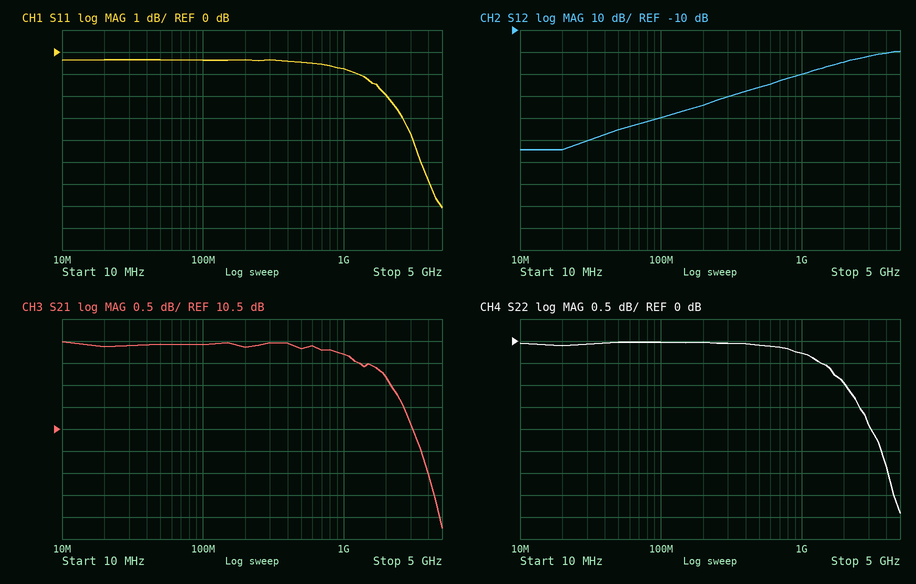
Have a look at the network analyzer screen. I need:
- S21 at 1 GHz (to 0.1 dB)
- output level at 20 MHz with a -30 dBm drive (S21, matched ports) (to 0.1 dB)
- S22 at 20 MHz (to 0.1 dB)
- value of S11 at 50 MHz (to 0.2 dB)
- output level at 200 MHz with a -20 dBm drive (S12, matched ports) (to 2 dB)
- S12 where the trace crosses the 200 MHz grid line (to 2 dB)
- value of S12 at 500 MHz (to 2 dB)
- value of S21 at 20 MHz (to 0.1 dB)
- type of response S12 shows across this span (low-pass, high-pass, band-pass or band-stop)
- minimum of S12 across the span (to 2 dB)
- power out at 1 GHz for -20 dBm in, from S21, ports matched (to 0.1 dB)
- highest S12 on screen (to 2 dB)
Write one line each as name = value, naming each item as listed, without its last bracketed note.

S21 at 1 GHz = 12.2 dB
output level at 20 MHz with a -30 dBm drive (S21, matched ports) = -17.6 dBm
S22 at 20 MHz = -0.1 dB
value of S11 at 50 MHz = -0.4 dB
output level at 200 MHz with a -20 dBm drive (S12, matched ports) = -64 dBm
S12 where the trace crosses the 200 MHz grid line = -44 dB
value of S12 at 500 MHz = -36 dB
value of S21 at 20 MHz = 12.4 dB
type of response S12 shows across this span = high-pass
minimum of S12 across the span = -64 dB
power out at 1 GHz for -20 dBm in, from S21, ports matched = -7.8 dBm
highest S12 on screen = -20 dB
